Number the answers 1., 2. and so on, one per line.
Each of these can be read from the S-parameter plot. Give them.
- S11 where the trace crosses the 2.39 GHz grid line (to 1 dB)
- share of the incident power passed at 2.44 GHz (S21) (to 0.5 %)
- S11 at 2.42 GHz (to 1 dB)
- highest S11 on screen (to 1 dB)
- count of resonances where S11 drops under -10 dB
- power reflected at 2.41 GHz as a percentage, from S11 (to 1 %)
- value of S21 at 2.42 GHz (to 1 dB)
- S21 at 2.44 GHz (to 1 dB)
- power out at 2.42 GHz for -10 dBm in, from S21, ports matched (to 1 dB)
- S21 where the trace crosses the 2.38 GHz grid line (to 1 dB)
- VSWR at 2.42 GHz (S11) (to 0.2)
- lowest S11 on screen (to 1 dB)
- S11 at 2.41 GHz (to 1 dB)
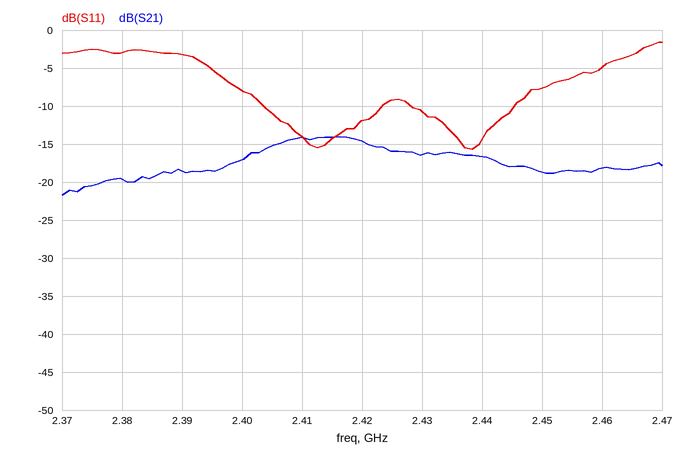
1. -3 dB
2. 2.0 %
3. -12 dB
4. -2 dB
5. 2
6. 4 %
7. -15 dB
8. -17 dB
9. -25 dBm
10. -20 dB
11. 1.6
12. -16 dB
13. -14 dB
